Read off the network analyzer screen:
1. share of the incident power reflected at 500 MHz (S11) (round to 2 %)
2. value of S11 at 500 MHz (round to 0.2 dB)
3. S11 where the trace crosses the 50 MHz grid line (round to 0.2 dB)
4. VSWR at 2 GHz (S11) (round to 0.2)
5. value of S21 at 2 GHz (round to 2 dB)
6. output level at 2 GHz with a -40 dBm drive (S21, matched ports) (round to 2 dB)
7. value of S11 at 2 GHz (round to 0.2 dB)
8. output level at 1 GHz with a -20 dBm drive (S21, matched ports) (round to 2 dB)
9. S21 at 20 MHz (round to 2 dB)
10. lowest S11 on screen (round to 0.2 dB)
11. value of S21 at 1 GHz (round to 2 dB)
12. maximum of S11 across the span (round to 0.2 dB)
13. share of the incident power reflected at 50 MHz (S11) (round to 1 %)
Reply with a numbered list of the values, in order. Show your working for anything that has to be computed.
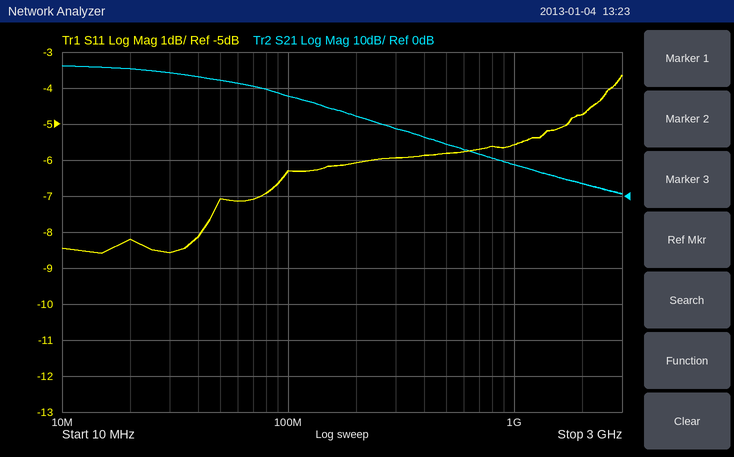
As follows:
1. 10^(-5.8/10) ≈ 26 %
2. -5.8 dB
3. -7.0 dB
4. |Γ| = 10^(-4.8/20) = 0.5754; VSWR = (1 + 0.5754)/(1 − 0.5754) ≈ 3.71, so 3.8 to the nearest 0.2
5. 4 dB
6. -40 dBm + (4 dB) = -36 dBm
7. -4.8 dB
8. -20 dBm + (8 dB) = -12 dBm
9. 36 dB
10. -8.6 dB
11. 8 dB
12. -3.6 dB
13. 10^(-7/10) ≈ 20 %
